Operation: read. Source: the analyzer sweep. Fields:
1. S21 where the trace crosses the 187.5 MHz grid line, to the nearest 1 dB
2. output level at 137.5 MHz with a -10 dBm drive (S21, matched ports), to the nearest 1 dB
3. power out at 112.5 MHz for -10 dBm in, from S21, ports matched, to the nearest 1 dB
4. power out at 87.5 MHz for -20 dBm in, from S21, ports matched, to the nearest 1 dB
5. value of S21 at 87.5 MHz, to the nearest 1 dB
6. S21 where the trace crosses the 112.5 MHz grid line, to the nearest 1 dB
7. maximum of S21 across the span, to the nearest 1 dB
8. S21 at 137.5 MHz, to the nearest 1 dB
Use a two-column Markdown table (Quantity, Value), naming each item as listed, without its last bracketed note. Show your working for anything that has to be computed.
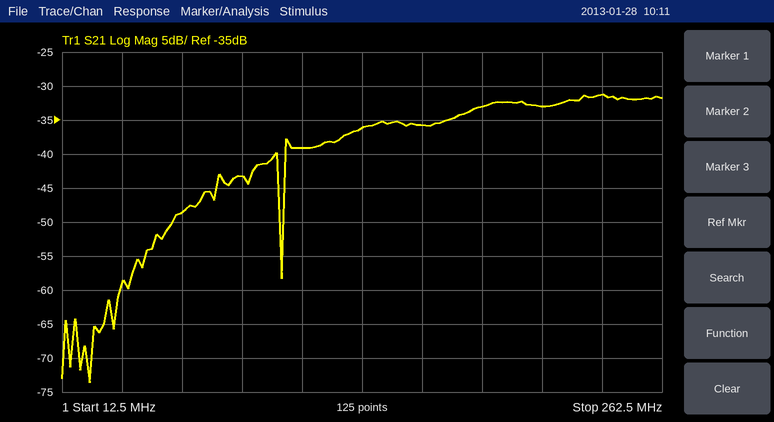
| Quantity | Value |
|---|---|
| S21 where the trace crosses the 187.5 MHz grid line, to the nearest 1 dB | -33 dB |
| output level at 137.5 MHz with a -10 dBm drive (S21, matched ports), to the nearest 1 dB | -10 dBm + (-36 dB) = -46 dBm |
| power out at 112.5 MHz for -10 dBm in, from S21, ports matched, to the nearest 1 dB | -10 dBm + (-39 dB) = -49 dBm |
| power out at 87.5 MHz for -20 dBm in, from S21, ports matched, to the nearest 1 dB | -20 dBm + (-43 dB) = -63 dBm |
| value of S21 at 87.5 MHz, to the nearest 1 dB | -43 dB |
| S21 where the trace crosses the 112.5 MHz grid line, to the nearest 1 dB | -39 dB |
| maximum of S21 across the span, to the nearest 1 dB | -31 dB |
| S21 at 137.5 MHz, to the nearest 1 dB | -36 dB |
